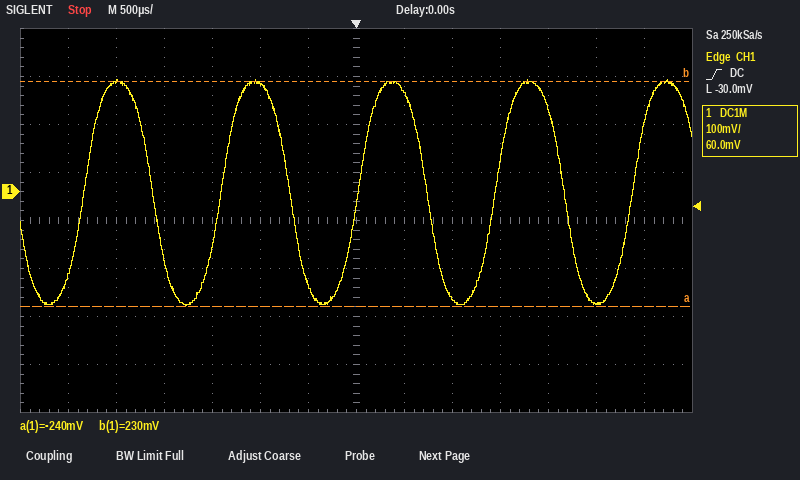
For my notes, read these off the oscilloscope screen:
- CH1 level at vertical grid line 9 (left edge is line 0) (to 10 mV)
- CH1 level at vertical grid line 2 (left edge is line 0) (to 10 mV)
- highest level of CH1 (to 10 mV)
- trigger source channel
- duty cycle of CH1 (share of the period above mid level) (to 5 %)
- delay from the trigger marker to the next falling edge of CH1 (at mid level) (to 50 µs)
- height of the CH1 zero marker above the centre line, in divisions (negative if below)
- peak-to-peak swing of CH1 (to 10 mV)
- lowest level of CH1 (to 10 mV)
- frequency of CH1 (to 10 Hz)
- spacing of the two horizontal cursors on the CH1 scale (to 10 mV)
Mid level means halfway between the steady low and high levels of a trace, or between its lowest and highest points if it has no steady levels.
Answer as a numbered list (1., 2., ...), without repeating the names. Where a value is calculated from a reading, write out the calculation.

1. -220 mV
2. 230 mV
3. 230 mV
4. CH1
5. 50 %
6. 750 µs
7. +0.6 div
8. 230 mV − (-240 mV) = 470 mV
9. -240 mV
10. 700 Hz
11. 470 mV
